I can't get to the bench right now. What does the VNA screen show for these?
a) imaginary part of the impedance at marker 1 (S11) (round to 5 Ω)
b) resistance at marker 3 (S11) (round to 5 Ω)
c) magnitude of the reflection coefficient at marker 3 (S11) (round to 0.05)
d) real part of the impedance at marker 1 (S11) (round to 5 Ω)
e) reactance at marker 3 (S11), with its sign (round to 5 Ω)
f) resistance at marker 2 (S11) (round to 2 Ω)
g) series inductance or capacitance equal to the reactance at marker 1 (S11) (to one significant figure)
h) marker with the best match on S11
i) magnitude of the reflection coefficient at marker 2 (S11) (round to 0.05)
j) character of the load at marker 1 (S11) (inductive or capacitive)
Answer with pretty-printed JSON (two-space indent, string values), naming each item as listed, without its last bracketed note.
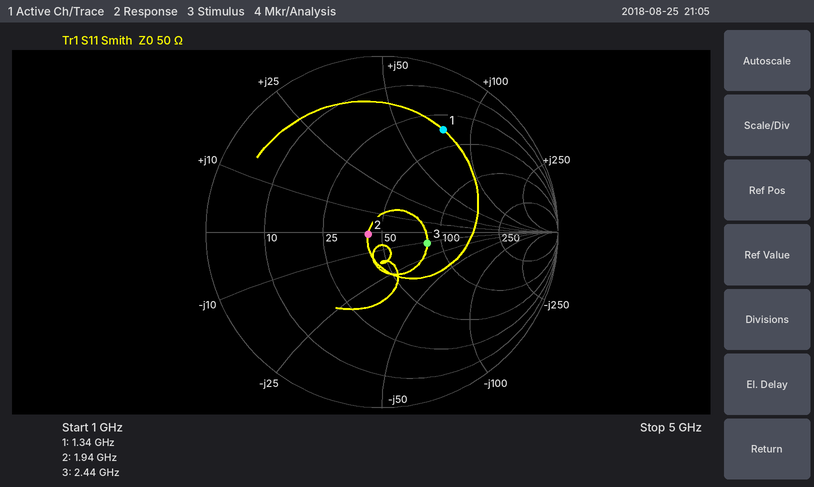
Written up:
{
  "imaginary part of the impedance at marker 1 (S11)": "+75 Ω",
  "resistance at marker 3 (S11)": "85 Ω",
  "magnitude of the reflection coefficient at marker 3 (S11)": "0.25",
  "real part of the impedance at marker 1 (S11)": "35 Ω",
  "reactance at marker 3 (S11), with its sign": "-10 Ω",
  "resistance at marker 2 (S11)": "42 Ω",
  "series inductance or capacitance equal to the reactance at marker 1 (S11)": "9 nH",
  "marker with the best match on S11": "marker 2",
  "magnitude of the reflection coefficient at marker 2 (S11)": "0.10",
  "character of the load at marker 1 (S11)": "inductive"
}
